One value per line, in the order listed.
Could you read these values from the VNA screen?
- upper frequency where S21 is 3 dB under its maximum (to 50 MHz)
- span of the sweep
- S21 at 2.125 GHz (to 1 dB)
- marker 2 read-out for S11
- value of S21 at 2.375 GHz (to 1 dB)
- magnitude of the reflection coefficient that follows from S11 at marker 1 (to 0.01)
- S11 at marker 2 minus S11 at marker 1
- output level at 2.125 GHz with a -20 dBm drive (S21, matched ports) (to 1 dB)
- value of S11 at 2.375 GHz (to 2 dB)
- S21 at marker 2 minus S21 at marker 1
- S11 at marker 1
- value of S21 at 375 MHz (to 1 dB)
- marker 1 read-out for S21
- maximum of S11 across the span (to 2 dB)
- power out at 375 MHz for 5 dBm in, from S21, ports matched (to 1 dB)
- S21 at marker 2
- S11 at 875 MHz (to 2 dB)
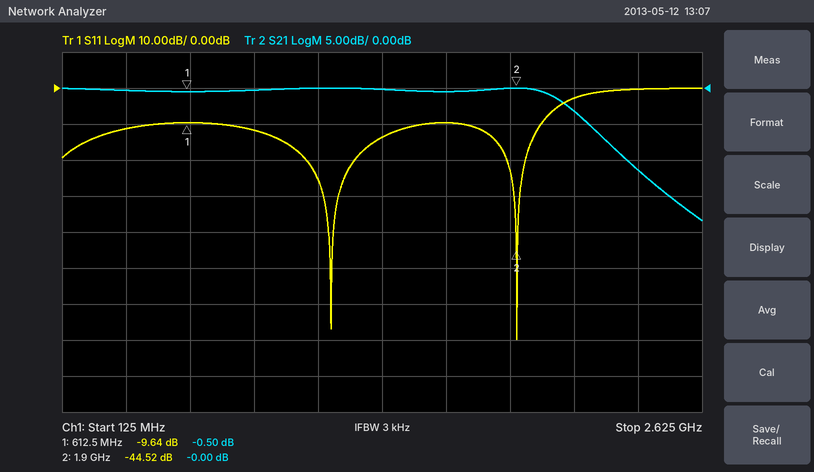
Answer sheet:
2.10 GHz
2.5 GHz
-3 dB
-44.52 dB
-11 dB
0.33
-34.88 dB
-23 dBm
0 dB
0.50 dB
-9.64 dB
0 dB
-0.50 dB
0 dB
5 dBm
-0.00 dB
-12 dB
